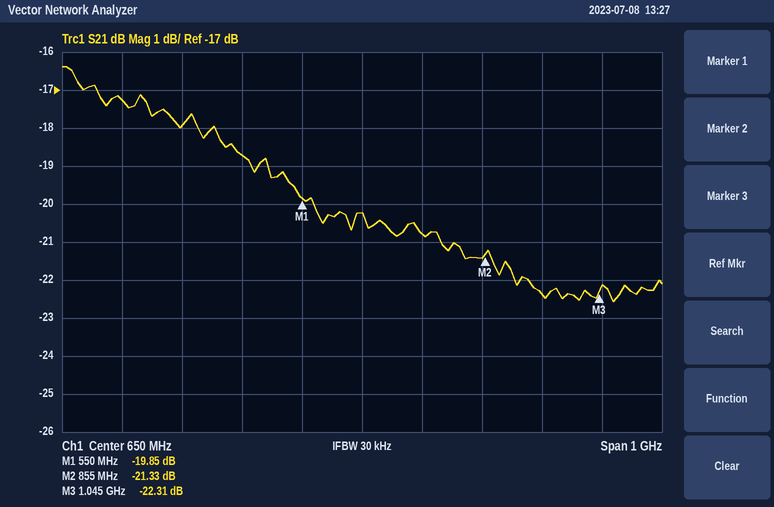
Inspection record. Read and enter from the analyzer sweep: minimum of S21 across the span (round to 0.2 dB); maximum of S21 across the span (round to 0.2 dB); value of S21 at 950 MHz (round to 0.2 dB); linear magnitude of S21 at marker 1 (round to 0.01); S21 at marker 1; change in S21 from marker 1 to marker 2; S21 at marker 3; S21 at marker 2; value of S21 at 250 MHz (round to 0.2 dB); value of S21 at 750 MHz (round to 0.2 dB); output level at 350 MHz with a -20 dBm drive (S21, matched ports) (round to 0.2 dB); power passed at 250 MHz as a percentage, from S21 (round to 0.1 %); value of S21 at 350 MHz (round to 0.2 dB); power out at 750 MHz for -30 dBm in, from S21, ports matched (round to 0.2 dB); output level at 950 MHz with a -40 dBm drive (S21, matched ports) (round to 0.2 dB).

-22.6 dB
-16.4 dB
-22.4 dB
0.10
-19.85 dB
-1.48 dB
-22.31 dB
-21.33 dB
-17.2 dB
-20.8 dB
-38.0 dBm
1.9 %
-18.0 dB
-50.8 dBm
-62.4 dBm
